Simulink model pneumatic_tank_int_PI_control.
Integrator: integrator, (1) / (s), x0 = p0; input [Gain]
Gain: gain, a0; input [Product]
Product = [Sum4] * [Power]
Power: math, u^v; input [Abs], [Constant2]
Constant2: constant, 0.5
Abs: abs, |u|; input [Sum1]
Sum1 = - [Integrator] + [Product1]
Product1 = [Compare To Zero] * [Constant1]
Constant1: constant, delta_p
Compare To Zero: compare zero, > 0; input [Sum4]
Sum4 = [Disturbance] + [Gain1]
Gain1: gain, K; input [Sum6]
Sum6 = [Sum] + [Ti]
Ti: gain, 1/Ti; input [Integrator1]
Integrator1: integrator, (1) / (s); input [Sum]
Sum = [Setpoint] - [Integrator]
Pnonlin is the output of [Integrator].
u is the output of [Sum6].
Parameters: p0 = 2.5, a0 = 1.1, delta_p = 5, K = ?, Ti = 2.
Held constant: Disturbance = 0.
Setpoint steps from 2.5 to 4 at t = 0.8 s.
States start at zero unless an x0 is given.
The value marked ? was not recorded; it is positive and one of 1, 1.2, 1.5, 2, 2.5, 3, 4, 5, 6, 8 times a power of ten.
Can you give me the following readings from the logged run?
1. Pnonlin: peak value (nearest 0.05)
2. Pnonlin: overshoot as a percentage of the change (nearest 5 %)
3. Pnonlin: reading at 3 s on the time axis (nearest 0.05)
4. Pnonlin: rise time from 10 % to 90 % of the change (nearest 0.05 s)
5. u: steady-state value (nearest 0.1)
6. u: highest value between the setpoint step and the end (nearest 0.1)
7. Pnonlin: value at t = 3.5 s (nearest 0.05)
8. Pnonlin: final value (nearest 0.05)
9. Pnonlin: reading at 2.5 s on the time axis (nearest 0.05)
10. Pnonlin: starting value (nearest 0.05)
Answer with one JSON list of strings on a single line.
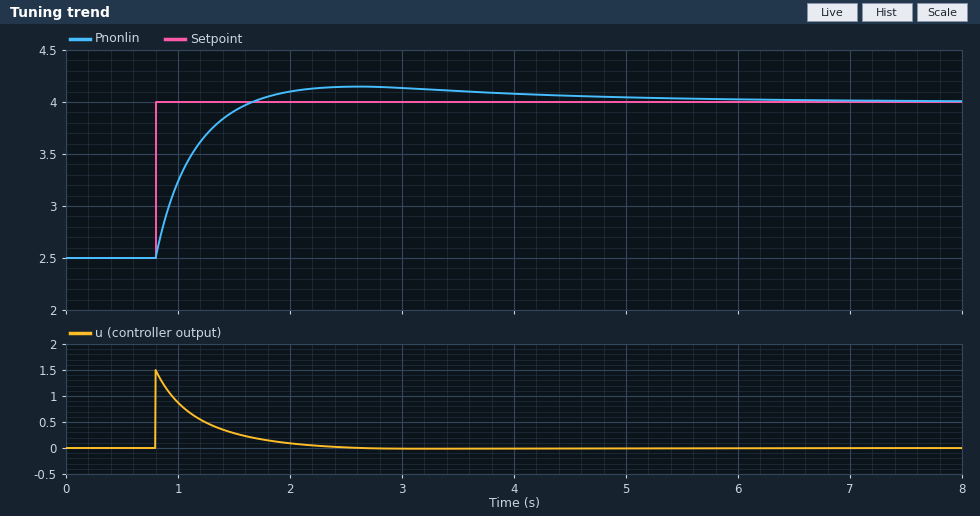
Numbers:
["4.15", "10 %", "4.15", "0.60 s", "0.0", "1.5", "4.10", "4.00", "4.15", "2.50"]
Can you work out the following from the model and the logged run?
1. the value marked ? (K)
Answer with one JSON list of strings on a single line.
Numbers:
["2"]
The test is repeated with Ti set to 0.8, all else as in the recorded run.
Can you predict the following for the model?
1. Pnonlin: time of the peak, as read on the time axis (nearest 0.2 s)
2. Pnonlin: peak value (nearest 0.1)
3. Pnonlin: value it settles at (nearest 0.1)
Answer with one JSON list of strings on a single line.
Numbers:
["2.2 s", "4.3", "4.0"]
